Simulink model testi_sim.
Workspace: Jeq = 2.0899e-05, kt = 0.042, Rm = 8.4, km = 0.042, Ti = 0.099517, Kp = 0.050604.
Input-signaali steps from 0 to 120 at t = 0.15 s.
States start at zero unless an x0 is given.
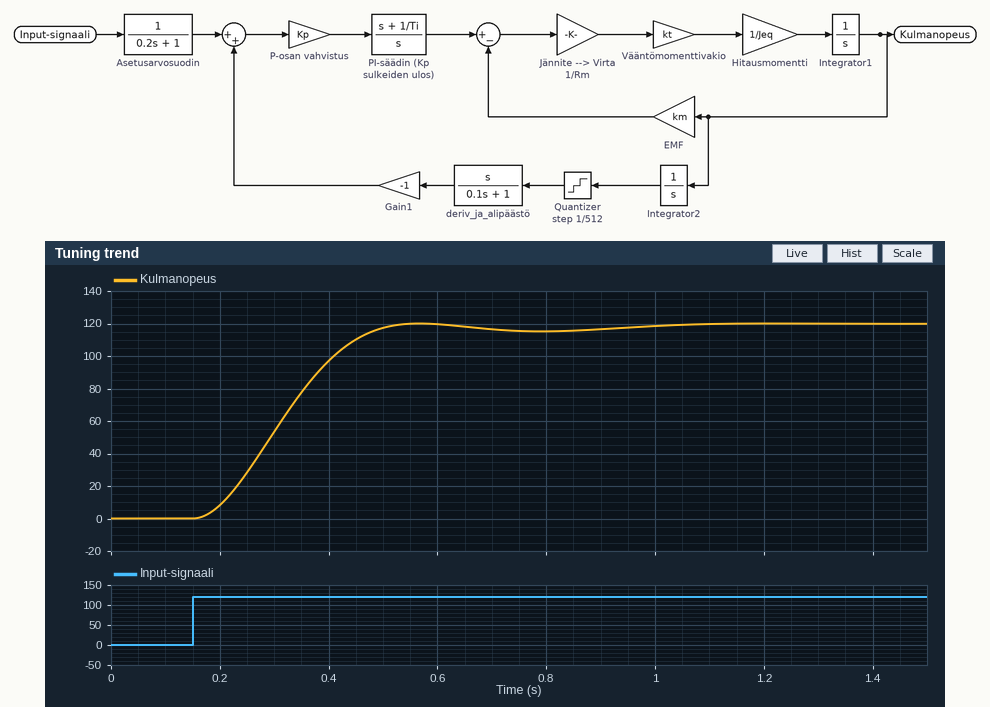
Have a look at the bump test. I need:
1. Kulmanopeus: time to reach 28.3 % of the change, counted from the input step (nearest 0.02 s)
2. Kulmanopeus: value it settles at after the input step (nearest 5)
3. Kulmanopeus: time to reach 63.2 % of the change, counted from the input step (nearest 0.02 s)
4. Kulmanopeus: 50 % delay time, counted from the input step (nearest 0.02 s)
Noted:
0.12 s
120
0.20 s
0.16 s
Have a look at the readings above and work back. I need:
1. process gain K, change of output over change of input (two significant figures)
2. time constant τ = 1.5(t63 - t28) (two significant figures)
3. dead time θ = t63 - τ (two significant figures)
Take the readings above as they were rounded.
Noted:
1.0
0.12 s
0.080 s
